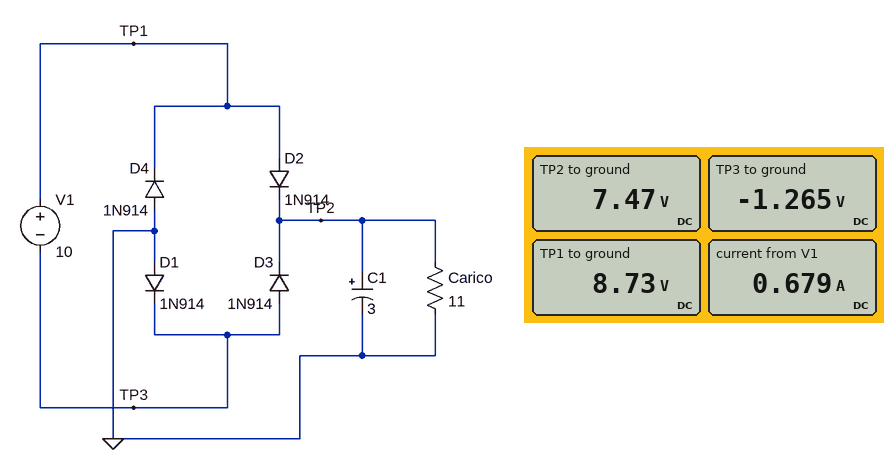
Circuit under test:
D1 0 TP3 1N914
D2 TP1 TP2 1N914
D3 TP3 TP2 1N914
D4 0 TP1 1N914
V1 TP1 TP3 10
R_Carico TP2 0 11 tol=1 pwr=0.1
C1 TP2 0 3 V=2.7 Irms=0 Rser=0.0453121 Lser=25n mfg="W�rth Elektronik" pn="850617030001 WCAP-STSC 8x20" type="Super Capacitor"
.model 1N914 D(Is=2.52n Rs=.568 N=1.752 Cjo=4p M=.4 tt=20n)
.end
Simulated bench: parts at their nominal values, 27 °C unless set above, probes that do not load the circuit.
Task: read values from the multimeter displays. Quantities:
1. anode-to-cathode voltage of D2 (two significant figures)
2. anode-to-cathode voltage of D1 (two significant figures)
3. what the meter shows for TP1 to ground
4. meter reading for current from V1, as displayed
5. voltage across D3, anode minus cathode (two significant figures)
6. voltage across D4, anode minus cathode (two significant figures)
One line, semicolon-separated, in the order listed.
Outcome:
1.3 V; 1.3 V; 8.73 V; 0.679 A; -8.7 V; -8.7 V
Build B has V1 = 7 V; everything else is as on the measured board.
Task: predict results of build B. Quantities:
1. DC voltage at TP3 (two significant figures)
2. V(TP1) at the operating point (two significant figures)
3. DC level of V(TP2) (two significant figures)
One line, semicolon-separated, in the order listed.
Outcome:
-1.1 V; 5.9 V; 4.8 V
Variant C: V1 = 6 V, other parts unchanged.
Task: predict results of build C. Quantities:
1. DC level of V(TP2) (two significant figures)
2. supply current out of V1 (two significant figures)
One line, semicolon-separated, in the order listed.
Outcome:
3.9 V; 350 mA
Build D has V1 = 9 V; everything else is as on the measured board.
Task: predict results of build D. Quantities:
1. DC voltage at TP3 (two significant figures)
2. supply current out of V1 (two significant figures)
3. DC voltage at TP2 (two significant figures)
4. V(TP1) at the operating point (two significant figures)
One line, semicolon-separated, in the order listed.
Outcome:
-1.2 V; 600 mA; 6.6 V; 7.8 V
